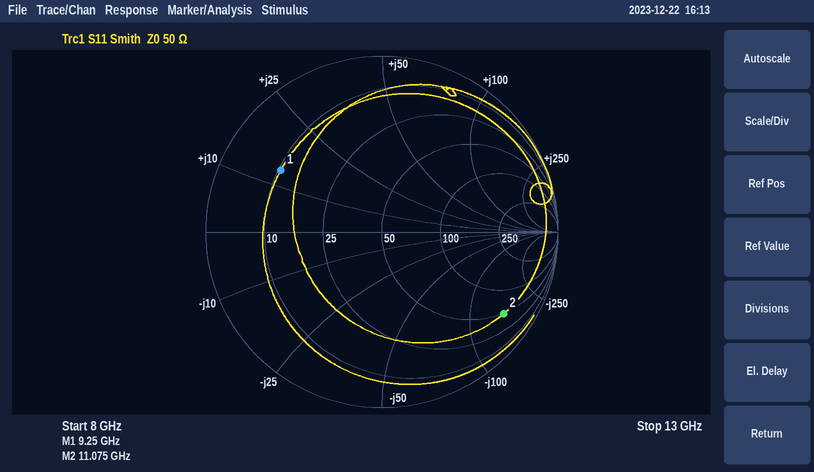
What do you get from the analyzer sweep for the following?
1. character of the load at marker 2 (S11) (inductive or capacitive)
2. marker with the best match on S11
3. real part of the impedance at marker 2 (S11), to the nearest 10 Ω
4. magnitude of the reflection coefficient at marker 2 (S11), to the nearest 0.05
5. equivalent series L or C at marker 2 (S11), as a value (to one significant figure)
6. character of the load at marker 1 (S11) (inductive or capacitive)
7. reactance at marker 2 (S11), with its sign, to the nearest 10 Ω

capacitive
marker 1
50 Ω
0.85
100 fF
inductive
-150 Ω
